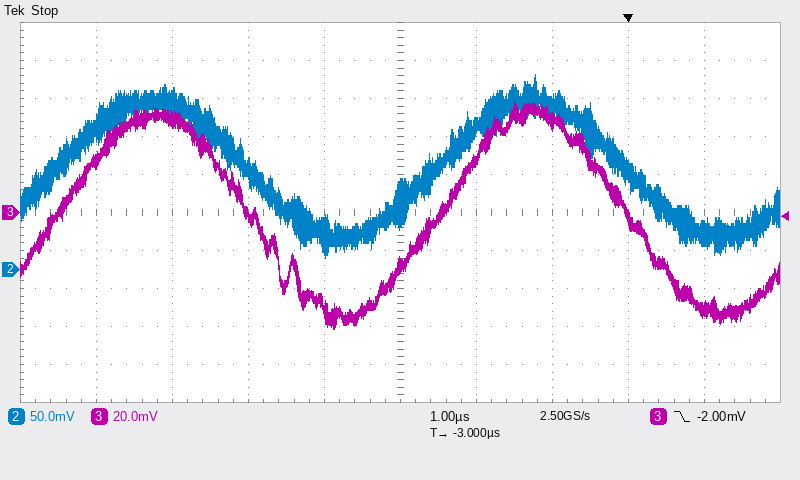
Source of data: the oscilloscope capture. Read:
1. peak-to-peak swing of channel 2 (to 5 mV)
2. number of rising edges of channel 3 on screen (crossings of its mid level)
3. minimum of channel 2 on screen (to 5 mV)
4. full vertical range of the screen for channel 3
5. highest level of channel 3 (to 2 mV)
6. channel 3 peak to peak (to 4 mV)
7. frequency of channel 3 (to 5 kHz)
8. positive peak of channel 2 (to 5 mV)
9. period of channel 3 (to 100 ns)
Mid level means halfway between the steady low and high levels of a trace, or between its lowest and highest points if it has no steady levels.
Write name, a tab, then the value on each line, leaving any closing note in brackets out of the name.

peak-to-peak swing of channel 2	240 mV
number of rising edges of channel 3 on screen	2
minimum of channel 2 on screen	15 mV
full vertical range of the screen for channel 3	200 mV
highest level of channel 3	58 mV
channel 3 peak to peak	120 mV
frequency of channel 3	200 kHz
positive peak of channel 2	255 mV
period of channel 3	5.0 µs
